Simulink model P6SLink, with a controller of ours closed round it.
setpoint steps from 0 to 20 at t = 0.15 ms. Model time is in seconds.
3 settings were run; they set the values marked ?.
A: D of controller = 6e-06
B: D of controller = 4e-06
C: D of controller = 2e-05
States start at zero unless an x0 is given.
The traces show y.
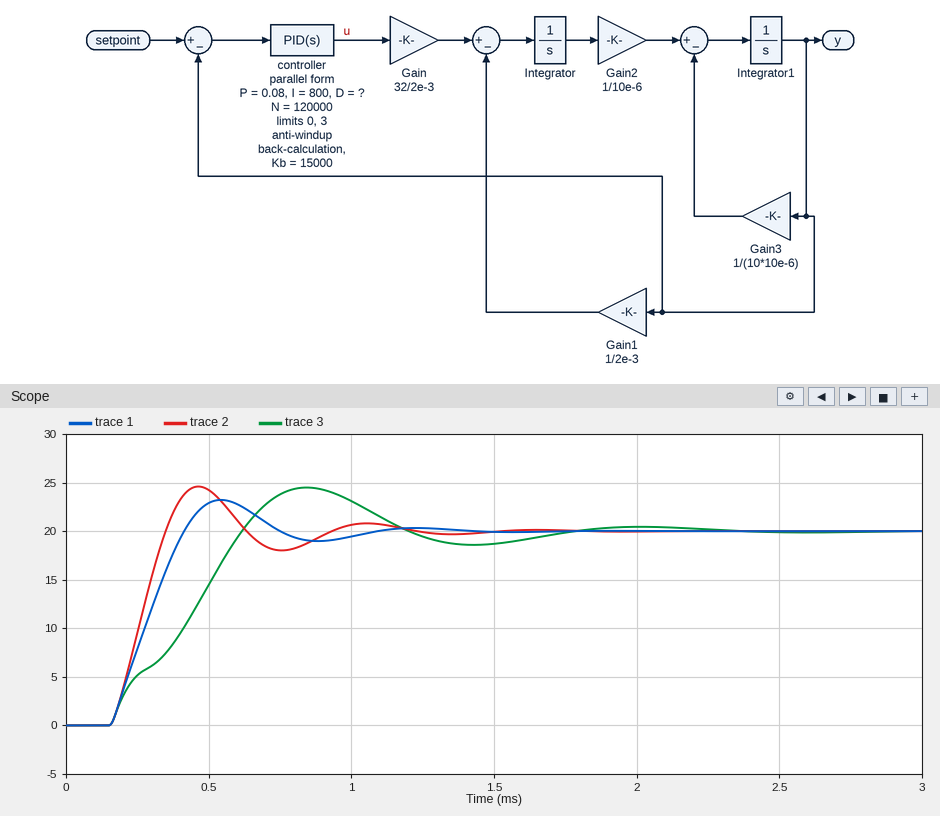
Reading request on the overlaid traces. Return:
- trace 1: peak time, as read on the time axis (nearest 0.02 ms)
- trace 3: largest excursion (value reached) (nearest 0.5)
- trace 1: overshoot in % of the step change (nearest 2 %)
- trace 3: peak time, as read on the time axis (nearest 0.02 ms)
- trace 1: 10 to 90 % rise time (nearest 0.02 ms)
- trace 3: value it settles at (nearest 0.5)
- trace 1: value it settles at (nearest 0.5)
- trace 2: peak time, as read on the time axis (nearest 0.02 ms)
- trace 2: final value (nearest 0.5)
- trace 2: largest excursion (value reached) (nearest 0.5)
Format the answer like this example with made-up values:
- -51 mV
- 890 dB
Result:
- 0.54 ms
- 24.5
- 16 %
- 0.84 ms
- 0.20 ms
- 20.0
- 20.0
- 0.46 ms
- 20.0
- 24.5
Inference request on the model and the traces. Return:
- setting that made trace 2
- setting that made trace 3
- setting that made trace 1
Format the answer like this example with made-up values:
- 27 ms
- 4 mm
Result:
- B
- C
- A
